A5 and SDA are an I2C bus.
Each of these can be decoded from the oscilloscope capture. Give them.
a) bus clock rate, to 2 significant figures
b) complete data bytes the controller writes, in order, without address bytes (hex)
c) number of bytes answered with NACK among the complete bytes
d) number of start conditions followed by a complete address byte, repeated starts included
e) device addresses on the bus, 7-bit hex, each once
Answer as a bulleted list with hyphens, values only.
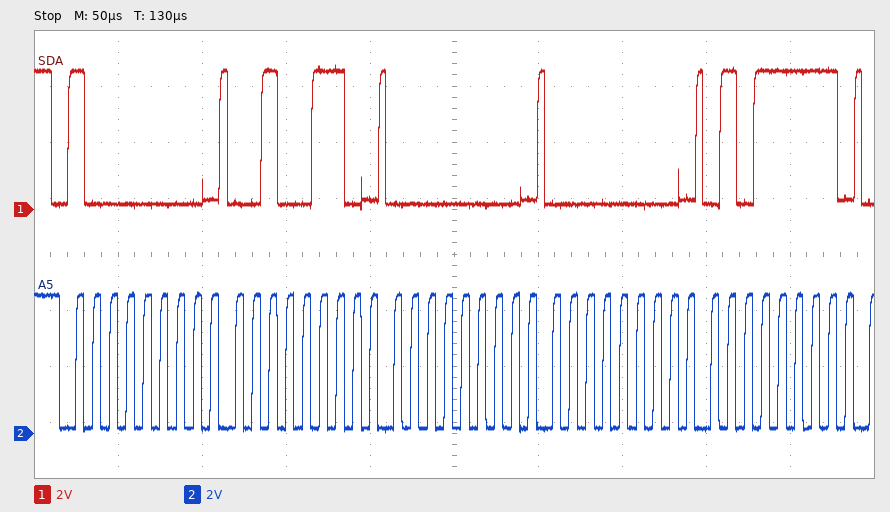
- 100 kHz
- 26 00 00 5F
- 0
- 1
- 0x40
